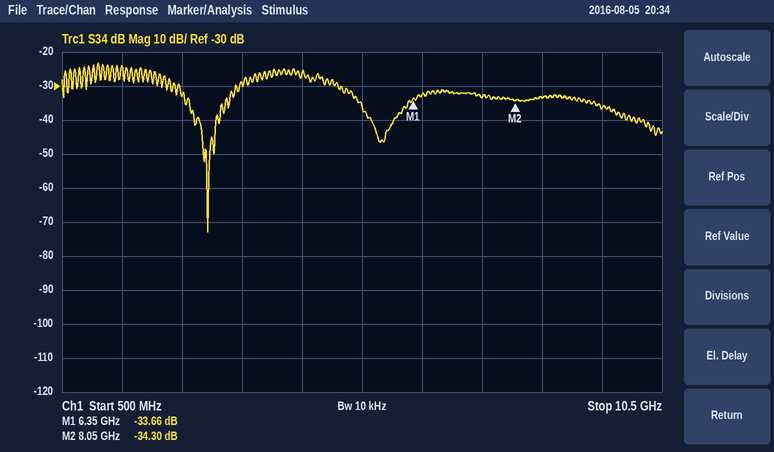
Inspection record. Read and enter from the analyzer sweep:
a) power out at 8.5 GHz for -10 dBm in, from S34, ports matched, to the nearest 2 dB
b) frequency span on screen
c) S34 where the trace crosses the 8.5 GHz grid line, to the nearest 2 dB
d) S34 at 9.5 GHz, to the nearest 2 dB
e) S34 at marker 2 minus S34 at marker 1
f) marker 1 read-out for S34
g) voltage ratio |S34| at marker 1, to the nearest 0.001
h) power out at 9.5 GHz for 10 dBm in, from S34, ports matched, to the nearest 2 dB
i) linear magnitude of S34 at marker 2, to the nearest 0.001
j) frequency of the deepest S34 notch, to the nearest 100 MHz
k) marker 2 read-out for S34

-44 dBm
10 GHz
-34 dB
-36 dB
-0.64 dB
-33.66 dB
0.021
-26 dBm
0.019
2.9 GHz
-34.30 dB
